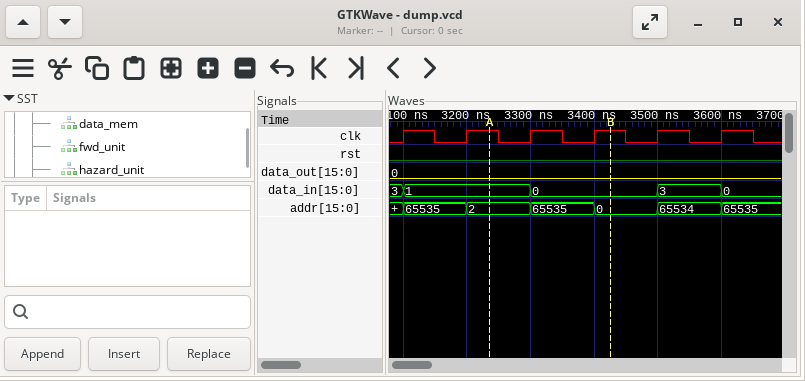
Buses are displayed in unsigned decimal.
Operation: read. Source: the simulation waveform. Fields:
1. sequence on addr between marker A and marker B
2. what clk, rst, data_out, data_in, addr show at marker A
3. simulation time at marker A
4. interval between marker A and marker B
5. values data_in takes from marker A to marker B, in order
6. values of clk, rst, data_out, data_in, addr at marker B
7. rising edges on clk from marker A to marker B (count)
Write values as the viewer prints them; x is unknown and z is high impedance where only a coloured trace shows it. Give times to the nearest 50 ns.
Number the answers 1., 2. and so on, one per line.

1. 2, 65535, 0
2. clk=1, rst=0, data_out=0, data_in=1, addr=2
3. 3250 ns
4. 200 ns
5. 1, 0
6. clk=1, rst=0, data_out=0, data_in=0, addr=0
7. 2
